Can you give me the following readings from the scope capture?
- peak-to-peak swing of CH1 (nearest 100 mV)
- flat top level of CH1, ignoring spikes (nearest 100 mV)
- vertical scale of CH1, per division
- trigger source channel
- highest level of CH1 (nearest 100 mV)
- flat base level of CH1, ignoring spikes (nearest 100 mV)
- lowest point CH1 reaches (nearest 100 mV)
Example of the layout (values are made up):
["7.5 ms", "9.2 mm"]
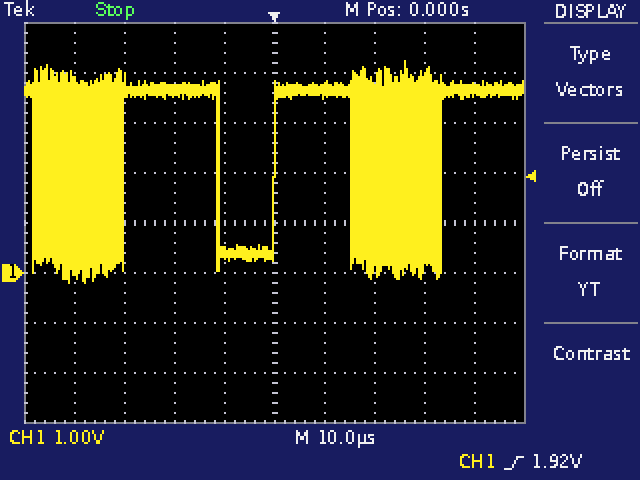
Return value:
["4.4 V", "3.7 V", "1 V", "CH1", "4.2 V", "400 mV", "-200 mV"]
